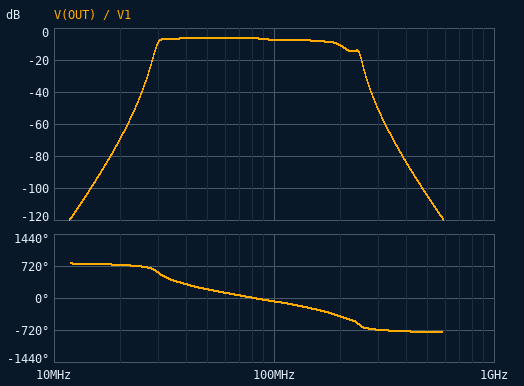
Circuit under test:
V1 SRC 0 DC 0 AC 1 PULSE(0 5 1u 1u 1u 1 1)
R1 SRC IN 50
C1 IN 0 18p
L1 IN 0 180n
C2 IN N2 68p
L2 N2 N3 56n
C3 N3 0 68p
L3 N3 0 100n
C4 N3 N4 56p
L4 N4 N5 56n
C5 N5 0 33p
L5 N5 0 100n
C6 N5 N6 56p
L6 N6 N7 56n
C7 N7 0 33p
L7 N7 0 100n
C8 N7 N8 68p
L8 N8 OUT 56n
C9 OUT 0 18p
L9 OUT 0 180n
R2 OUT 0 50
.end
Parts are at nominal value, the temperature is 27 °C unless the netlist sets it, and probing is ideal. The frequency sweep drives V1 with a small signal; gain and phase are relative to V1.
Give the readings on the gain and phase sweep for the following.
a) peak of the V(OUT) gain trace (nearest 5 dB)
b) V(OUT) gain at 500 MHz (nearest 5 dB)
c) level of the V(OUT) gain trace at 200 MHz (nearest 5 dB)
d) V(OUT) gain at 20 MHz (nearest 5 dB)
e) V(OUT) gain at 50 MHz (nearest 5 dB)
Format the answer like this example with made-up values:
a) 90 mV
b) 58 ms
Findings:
a) -5 dB
b) -105 dB
c) -10 dB
d) -70 dB
e) -5 dB
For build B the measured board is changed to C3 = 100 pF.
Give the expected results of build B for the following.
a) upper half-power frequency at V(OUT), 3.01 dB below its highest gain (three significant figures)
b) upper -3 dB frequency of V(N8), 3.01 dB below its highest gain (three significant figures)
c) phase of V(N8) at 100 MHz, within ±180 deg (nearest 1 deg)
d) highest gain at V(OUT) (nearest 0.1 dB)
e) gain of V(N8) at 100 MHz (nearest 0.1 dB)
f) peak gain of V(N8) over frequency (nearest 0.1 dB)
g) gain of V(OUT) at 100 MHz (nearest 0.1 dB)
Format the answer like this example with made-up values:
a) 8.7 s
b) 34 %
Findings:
a) 96.0 MHz
b) 88.9 MHz
c) -54 deg
d) -6.3 dB
e) -8.3 dB
f) -4.2 dB
g) -9.6 dB
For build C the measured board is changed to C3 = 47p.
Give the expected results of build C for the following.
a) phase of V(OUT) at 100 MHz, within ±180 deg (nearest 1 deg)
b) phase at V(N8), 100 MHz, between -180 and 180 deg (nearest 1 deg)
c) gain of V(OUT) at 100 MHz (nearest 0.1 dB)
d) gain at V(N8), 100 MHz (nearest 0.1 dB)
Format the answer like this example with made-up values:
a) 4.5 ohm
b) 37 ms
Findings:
a) -61 deg
b) -23 deg
c) -6.4 dB
d) -5.2 dB
